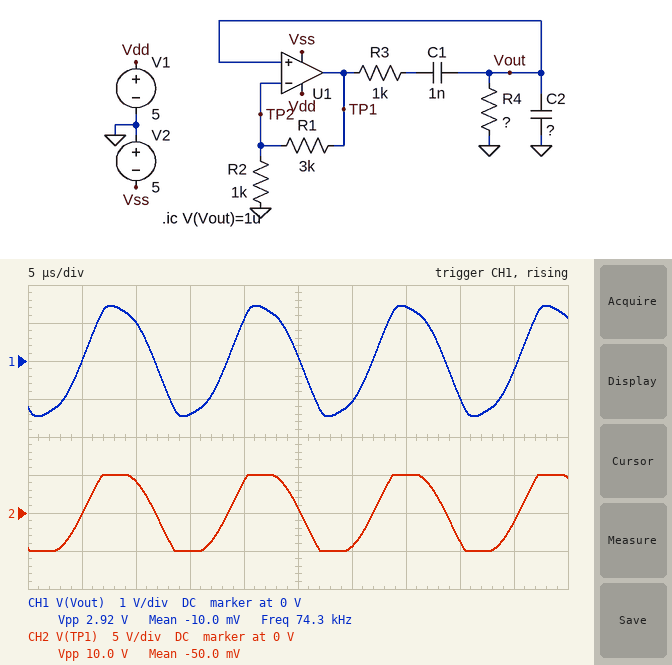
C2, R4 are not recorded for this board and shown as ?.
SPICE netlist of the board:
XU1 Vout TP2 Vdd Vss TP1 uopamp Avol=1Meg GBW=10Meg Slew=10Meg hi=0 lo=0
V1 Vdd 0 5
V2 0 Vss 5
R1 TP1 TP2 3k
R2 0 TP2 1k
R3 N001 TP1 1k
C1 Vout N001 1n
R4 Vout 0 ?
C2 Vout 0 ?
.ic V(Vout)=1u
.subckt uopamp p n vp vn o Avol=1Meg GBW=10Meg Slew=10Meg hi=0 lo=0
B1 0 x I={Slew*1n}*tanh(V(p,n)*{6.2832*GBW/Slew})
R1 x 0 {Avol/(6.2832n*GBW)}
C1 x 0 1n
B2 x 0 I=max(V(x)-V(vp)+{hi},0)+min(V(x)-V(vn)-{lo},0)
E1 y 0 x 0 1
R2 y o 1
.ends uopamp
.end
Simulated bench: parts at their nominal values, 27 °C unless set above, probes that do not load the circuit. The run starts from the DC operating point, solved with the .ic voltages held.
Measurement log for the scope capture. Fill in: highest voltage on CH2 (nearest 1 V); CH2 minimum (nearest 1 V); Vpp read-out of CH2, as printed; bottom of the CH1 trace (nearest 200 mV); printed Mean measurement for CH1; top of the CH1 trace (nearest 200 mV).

5 V
-5 V
10.0 V
-1.4 V
-10.0 mV
1.4 V
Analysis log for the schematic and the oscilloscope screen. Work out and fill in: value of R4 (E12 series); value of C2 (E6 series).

1.8 kΩ
2.2 nF
